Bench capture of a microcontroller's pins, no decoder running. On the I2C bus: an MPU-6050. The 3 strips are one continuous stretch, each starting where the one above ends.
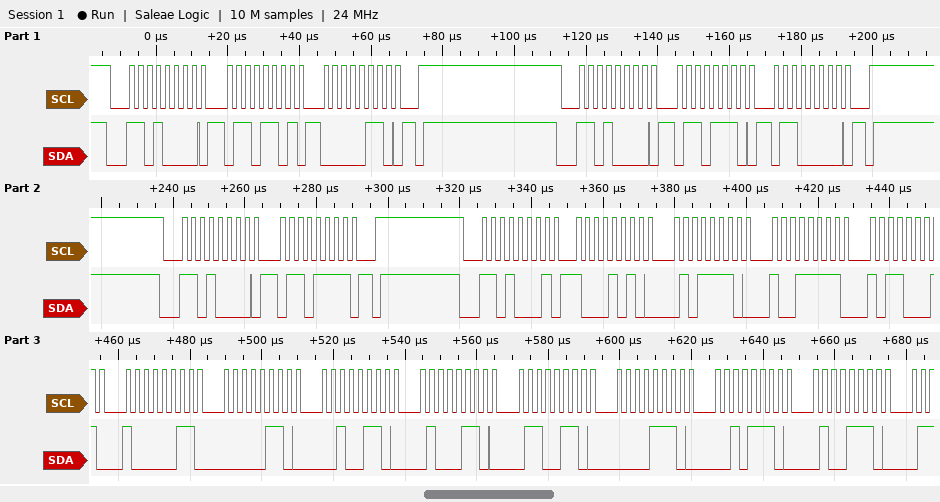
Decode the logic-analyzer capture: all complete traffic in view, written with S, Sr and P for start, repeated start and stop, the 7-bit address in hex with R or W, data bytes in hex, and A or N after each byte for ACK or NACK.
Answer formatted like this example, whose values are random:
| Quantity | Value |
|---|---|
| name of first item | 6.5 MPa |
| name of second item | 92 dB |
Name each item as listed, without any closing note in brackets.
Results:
| Quantity | Value |
|---|---|
| all complete traffic in view, written with S, Sr and P for start, repeated start and stop, the 7-bit address in hex with R or W, data bytes in hex, and A or N after each byte for ACK or NACK | S 68W A 6D A 06 A P S 68W A 6E A 60 A P S 68W A 6F A P S 68R A 8A A 5E A 9F A B1 A 83 A 06 A 26 A 46 A 66 A 0E A 2E A 4E A |
